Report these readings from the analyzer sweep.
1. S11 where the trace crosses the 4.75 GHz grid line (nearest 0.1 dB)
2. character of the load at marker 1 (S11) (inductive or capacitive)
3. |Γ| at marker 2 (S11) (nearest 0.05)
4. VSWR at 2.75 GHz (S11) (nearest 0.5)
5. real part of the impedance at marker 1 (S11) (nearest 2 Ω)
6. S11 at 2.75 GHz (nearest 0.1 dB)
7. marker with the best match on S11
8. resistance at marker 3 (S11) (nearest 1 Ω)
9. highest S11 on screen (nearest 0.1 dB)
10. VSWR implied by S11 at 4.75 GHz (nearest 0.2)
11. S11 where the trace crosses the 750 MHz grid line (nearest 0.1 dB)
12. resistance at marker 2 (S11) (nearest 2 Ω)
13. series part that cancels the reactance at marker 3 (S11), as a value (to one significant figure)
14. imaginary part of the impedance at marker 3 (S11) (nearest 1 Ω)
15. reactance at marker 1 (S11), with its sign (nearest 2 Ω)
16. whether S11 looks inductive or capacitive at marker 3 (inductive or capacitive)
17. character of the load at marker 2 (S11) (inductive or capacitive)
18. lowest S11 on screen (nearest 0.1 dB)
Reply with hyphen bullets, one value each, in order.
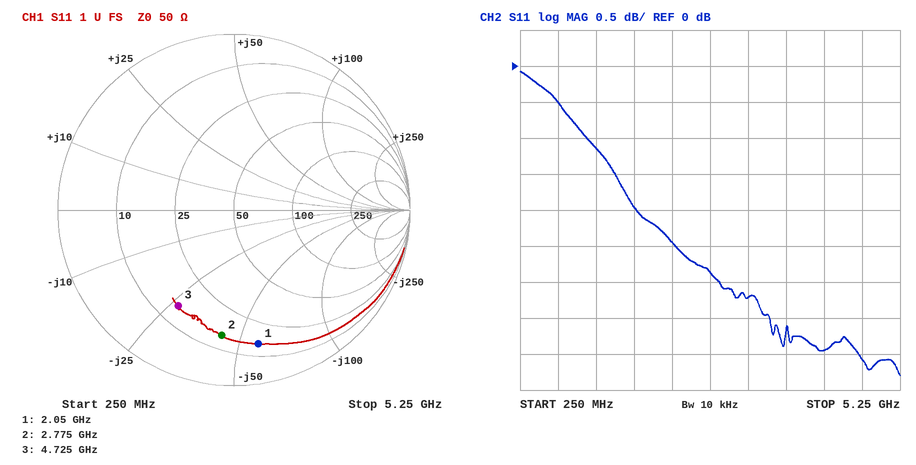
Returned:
- -4.1 dB
- capacitive
- 0.70
- 6.0
- 16 Ω
- -2.9 dB
- marker 3
- 15 Ω
- -0.1 dB
- 4.4
- -0.5 dB
- 14 Ω
- 900 pH
- -27 Ω
- -58 Ω
- capacitive
- capacitive
- -4.3 dB
